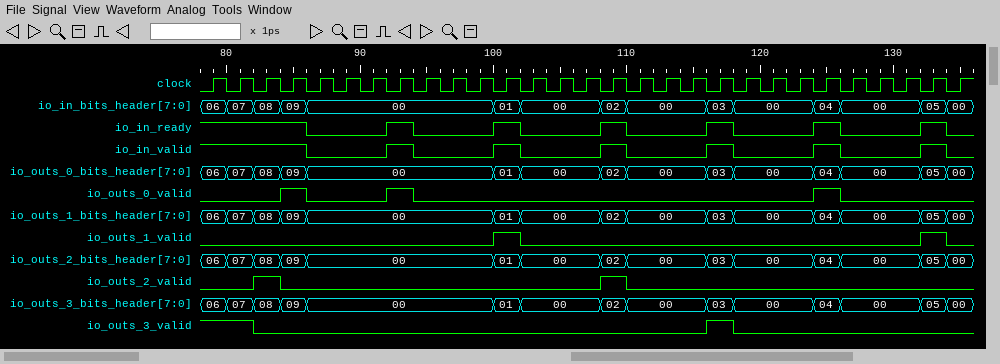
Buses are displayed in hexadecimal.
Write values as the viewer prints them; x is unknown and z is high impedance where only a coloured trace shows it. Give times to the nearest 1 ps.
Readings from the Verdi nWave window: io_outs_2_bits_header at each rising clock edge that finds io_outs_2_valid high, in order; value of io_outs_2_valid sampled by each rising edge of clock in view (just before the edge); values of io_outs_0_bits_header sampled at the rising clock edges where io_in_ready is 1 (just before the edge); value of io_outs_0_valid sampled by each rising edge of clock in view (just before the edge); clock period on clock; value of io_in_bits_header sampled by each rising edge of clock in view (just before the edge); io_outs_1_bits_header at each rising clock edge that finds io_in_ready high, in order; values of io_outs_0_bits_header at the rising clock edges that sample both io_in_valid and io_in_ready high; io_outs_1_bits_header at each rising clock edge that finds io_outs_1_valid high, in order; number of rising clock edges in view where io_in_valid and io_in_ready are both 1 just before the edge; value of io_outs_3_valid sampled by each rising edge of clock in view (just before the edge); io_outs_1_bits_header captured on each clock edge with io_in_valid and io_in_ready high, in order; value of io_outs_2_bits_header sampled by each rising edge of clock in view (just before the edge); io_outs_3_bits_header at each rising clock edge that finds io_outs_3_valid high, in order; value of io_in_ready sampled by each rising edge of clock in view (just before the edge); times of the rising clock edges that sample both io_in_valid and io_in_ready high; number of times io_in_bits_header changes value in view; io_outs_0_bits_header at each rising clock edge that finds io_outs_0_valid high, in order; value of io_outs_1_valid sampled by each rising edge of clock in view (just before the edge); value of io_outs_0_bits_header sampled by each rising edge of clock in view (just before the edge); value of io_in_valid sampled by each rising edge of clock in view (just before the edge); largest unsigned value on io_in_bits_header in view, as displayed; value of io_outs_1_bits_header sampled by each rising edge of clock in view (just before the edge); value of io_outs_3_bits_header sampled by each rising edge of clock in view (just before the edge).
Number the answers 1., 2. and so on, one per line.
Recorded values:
1. 08, 02
2. 0 0 1 0 0 0 0 0 0 0 0 0 0 0 0 1 0 0 0 0 0 0 0 0 0 0 0 0 0
3. 06, 07, 08, 09, 00, 01, 02, 03, 04, 05
4. 0 0 0 1 0 0 0 1 0 0 0 0 0 0 0 0 0 0 0 0 0 0 0 1 0 0 0 0 0
5. 2 ps
6. 06, 07, 08, 09, 00, 00, 00, 00, 00, 00, 00, 01, 00, 00, 00, 02, 00, 00, 00, 03, 00, 00, 00, 04, 00, 00, 00, 05, 00
7. 06, 07, 08, 09, 00, 01, 02, 03, 04, 05
8. 06, 07, 08, 09, 00, 01, 02, 03, 04, 05
9. 01, 05
10. 10
11. 1 1 0 0 0 0 0 0 0 0 0 0 0 0 0 0 0 0 0 1 0 0 0 0 0 0 0 0 0
12. 06, 07, 08, 09, 00, 01, 02, 03, 04, 05
13. 06, 07, 08, 09, 00, 00, 00, 00, 00, 00, 00, 01, 00, 00, 00, 02, 00, 00, 00, 03, 00, 00, 00, 04, 00, 00, 00, 05, 00
14. 06, 07, 03
15. 1 1 1 1 0 0 0 1 0 0 0 1 0 0 0 1 0 0 0 1 0 0 0 1 0 0 0 1 0
16. 79 ps, 81 ps, 83 ps, 85 ps, 93 ps, 101 ps, 109 ps, 117 ps, 125 ps, 133 ps
17. 14
18. 09, 00, 04
19. 0 0 0 0 0 0 0 0 0 0 0 1 0 0 0 0 0 0 0 0 0 0 0 0 0 0 0 1 0
20. 06, 07, 08, 09, 00, 00, 00, 00, 00, 00, 00, 01, 00, 00, 00, 02, 00, 00, 00, 03, 00, 00, 00, 04, 00, 00, 00, 05, 00
21. 1 1 1 1 0 0 0 1 0 0 0 1 0 0 0 1 0 0 0 1 0 0 0 1 0 0 0 1 0
22. 09
23. 06, 07, 08, 09, 00, 00, 00, 00, 00, 00, 00, 01, 00, 00, 00, 02, 00, 00, 00, 03, 00, 00, 00, 04, 00, 00, 00, 05, 00
24. 06, 07, 08, 09, 00, 00, 00, 00, 00, 00, 00, 01, 00, 00, 00, 02, 00, 00, 00, 03, 00, 00, 00, 04, 00, 00, 00, 05, 00
